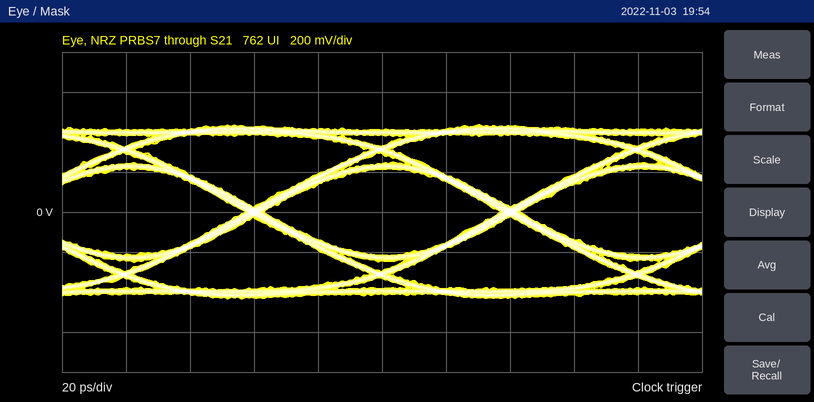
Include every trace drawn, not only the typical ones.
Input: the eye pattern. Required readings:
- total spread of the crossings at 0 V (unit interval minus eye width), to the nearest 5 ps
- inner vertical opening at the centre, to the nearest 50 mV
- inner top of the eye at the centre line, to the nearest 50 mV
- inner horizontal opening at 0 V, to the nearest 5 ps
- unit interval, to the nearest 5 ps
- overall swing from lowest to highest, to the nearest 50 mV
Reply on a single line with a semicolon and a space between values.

5 ps; 450 mV; 200 mV; 75 ps; 80 ps; 850 mV
